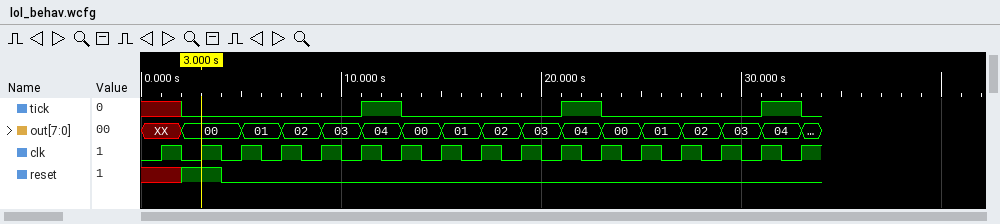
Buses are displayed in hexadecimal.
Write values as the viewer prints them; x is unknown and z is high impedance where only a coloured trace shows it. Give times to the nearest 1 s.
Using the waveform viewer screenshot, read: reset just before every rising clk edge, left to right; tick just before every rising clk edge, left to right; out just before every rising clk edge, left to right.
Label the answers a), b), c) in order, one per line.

a) x 1 0 0 0 0 0 0 0 0 0 0 0 0 0 0 0
b) x 0 0 0 0 0 1 0 0 0 0 1 0 0 0 0 1
c) XX, 00, 00, 01, 02, 03, 04, 00, 01, 02, 03, 04, 00, 01, 02, 03, 04
